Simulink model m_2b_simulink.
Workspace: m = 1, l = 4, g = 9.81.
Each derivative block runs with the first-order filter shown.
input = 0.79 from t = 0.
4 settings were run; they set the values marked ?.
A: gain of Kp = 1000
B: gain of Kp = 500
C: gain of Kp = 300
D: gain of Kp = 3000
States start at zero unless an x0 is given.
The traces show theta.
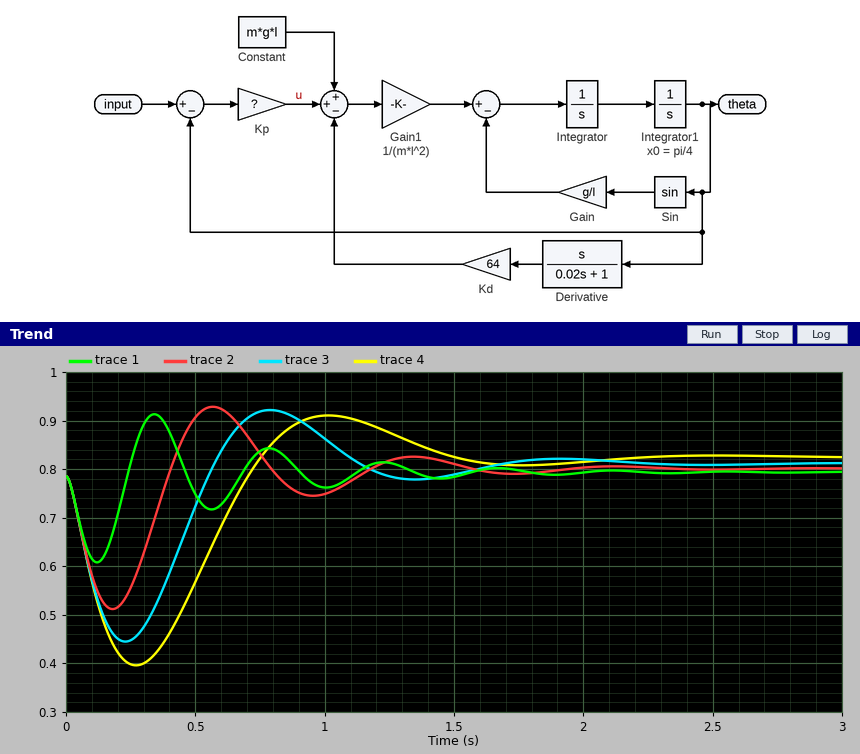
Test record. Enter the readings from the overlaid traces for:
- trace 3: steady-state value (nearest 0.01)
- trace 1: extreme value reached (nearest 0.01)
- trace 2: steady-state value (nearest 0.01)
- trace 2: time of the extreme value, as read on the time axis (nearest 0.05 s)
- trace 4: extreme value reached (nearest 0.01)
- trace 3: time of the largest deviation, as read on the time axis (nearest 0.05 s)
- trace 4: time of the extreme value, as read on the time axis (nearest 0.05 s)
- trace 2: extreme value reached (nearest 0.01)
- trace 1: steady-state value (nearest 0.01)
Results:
0.81
0.61
0.80
0.20 s
0.40
0.25 s
0.25 s
0.51
0.79
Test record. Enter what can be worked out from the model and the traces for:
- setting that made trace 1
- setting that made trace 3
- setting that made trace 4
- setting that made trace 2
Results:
D
B
C
A
